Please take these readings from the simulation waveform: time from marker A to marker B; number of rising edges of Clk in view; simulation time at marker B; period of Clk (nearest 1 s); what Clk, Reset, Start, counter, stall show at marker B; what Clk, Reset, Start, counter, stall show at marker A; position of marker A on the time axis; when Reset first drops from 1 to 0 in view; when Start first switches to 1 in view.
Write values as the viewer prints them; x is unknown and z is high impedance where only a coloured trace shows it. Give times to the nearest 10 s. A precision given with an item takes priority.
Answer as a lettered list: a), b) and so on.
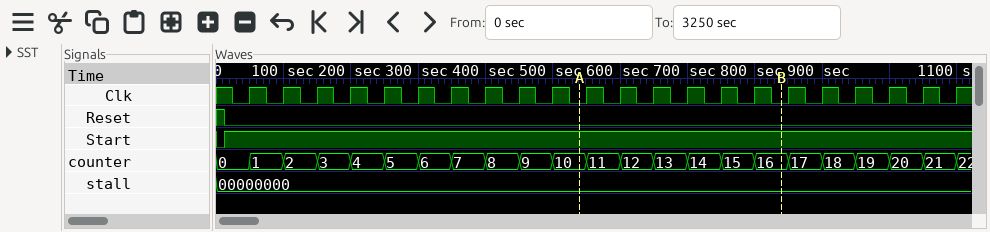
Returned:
a) 300 s
b) 22
c) 840 s
d) 50 s
e) Clk=0, Reset=0, Start=1, counter=16, stall=00000000
f) Clk=0, Reset=0, Start=1, counter=10, stall=00000000
g) 540 s
h) 10 s
i) 10 s
